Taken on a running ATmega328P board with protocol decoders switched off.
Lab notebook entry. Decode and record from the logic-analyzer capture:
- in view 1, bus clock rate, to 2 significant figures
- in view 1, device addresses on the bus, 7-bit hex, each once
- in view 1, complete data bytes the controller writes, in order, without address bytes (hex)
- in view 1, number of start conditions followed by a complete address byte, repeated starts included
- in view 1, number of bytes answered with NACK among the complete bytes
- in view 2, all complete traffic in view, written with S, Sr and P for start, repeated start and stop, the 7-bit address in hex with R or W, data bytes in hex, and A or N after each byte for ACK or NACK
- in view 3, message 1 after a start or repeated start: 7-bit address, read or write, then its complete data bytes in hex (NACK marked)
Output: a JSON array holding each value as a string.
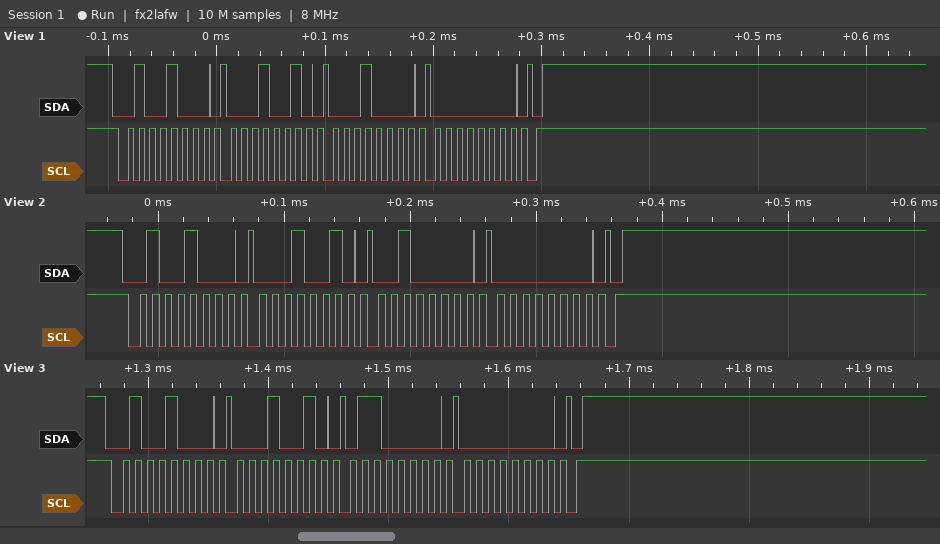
["100 kHz", "0x24", "12 10 00", "1", "0", "S 24W A 12 A 20 A 00 A P", "0x24 write: 12 60 00"]
